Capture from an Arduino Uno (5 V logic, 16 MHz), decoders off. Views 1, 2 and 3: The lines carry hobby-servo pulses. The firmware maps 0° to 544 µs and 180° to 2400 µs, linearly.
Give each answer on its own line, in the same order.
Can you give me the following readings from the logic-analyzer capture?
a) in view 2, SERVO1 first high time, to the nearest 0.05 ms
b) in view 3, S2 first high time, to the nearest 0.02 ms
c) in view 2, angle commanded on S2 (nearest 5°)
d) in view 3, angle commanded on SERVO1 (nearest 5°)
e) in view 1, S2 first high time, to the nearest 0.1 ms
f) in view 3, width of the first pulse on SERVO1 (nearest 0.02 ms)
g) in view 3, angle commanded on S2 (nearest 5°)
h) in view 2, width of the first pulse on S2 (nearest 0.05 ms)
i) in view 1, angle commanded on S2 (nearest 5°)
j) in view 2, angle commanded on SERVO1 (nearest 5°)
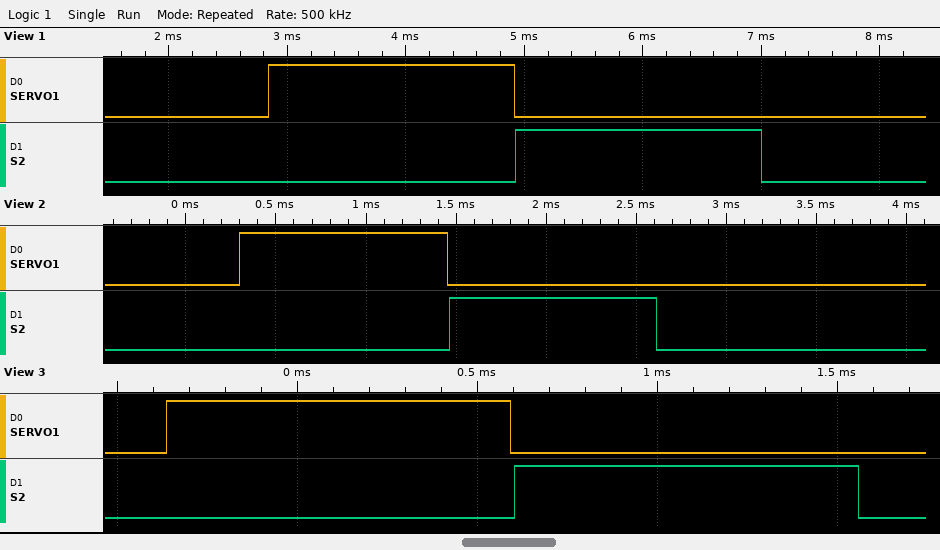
1.15 ms
0.96 ms
60°
40°
2.1 ms
0.96 ms
40°
1.15 ms
150°
60°
